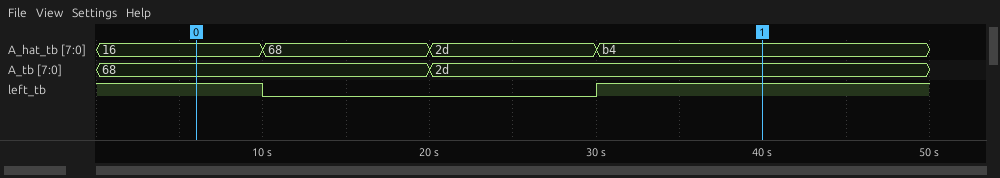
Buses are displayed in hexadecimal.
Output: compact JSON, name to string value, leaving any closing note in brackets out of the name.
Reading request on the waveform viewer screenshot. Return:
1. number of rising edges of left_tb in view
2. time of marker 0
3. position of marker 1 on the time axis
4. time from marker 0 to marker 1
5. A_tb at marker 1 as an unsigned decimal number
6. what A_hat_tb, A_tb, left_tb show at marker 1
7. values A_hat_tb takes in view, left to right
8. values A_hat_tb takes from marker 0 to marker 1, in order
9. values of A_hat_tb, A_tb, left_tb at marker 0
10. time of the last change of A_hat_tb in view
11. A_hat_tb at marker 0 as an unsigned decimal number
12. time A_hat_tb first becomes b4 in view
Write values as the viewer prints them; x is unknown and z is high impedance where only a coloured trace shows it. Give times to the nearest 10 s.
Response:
{"number of rising edges of left_tb in view": "1", "time of marker 0": "10 s", "position of marker 1 on the time axis": "40 s", "time from marker 0 to marker 1": "30 s", "A_tb at marker 1 as an unsigned decimal number": "45", "what A_hat_tb, A_tb, left_tb show at marker 1": "A_hat_tb=b4, A_tb=2d, left_tb=1", "values A_hat_tb takes in view, left to right": "16, 68, 2d, b4", "values A_hat_tb takes from marker 0 to marker 1, in order": "16, 68, 2d, b4", "values of A_hat_tb, A_tb, left_tb at marker 0": "A_hat_tb=16, A_tb=68, left_tb=1", "time of the last change of A_hat_tb in view": "30 s", "A_hat_tb at marker 0 as an unsigned decimal number": "22", "time A_hat_tb first becomes b4 in view": "30 s"}
